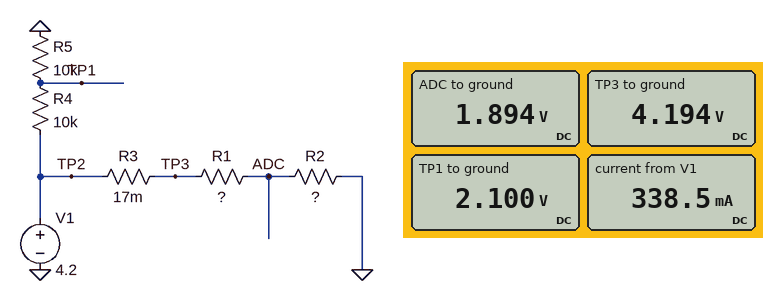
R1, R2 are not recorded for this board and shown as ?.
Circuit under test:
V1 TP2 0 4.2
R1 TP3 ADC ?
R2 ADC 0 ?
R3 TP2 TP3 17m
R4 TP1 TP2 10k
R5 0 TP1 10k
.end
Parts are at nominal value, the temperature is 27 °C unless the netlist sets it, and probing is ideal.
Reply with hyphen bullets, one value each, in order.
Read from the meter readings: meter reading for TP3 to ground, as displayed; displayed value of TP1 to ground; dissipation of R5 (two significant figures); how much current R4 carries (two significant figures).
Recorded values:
- 4.194 V
- 2.100 V
- 440 µW
- 210 µA
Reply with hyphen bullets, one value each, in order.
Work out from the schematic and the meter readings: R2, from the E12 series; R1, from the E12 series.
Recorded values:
- 5.6 Ω
- 6.8 Ω
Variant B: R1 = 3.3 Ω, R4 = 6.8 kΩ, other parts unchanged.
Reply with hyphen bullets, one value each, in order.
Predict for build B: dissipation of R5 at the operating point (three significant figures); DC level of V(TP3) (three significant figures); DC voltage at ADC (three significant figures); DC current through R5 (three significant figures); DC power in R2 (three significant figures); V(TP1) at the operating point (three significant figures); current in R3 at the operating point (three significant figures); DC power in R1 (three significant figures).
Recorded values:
- 625 µW
- 4.19 V
- 2.64 V
- 250 µA
- 1.24 W
- 2.50 V
- 471 mA
- 732 mW
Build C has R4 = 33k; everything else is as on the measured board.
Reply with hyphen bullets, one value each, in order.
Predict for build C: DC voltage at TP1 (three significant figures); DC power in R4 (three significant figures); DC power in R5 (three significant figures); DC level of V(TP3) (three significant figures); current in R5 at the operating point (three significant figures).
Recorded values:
- 977 mV
- 315 µW
- 95.4 µW
- 4.19 V
- 97.7 µA
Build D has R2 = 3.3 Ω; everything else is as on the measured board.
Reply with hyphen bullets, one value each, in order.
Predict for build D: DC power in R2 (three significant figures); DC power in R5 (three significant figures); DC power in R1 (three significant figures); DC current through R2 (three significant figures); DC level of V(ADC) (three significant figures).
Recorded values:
- 569 mW
- 441 µW
- 1.17 W
- 415 mA
- 1.37 V
